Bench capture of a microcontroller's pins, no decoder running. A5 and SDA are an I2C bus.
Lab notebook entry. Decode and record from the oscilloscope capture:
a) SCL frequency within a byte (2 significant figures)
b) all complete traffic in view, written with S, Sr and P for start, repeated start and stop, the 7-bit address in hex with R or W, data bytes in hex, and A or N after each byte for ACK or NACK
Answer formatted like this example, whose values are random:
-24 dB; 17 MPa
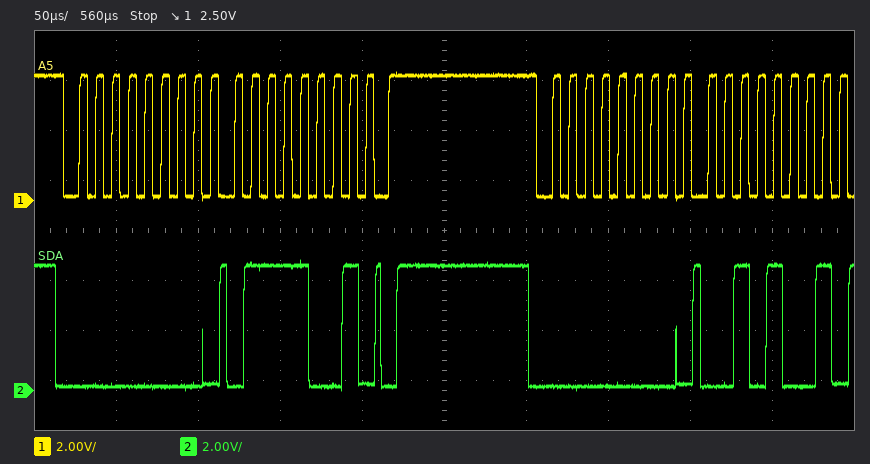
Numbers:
100 kHz; S 00W A 79 A P S 00W A 29 A
